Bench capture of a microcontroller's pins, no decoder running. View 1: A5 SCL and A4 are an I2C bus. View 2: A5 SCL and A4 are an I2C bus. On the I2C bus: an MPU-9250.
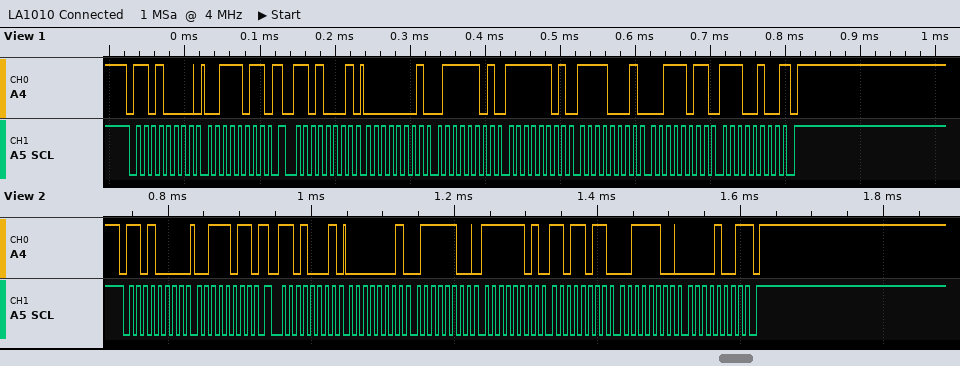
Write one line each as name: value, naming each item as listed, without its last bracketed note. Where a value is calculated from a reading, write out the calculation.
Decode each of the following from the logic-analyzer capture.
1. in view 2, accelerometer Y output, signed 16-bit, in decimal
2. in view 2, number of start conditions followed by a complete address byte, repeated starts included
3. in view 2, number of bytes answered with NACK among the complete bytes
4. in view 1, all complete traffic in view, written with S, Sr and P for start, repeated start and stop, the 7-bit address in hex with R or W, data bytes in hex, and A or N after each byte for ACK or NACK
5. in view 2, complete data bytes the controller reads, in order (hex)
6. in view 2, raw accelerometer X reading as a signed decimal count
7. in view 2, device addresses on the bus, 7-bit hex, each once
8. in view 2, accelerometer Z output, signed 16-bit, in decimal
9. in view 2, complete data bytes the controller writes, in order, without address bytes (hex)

in view 2, accelerometer Y output, signed 16-bit, in decimal: 0xFDDB = -549
in view 2, number of start conditions followed by a complete address byte, repeated starts included: 2
in view 2, number of bytes answered with NACK among the complete bytes: 1
in view 1, all complete traffic in view, written with S, Sr and P for start, repeated start and stop, the 7-bit address in hex with R or W, data bytes in hex, and A or N after each byte for ACK or NACK: S 68W A 3B A Sr 68R A 01 A 7D A FD A F1 A 3B A E4 N P
in view 2, complete data bytes the controller reads, in order: 01 7C FD DB 3C 09
in view 2, raw accelerometer X reading as a signed decimal count: 0x017C = 380
in view 2, device addresses on the bus, 7-bit hex, each once: 0x68
in view 2, accelerometer Z output, signed 16-bit, in decimal: 0x3C09 = 15369
in view 2, complete data bytes the controller writes, in order, without address bytes: 3B
